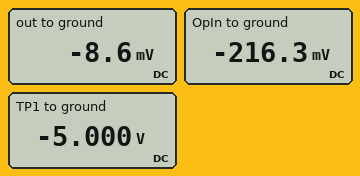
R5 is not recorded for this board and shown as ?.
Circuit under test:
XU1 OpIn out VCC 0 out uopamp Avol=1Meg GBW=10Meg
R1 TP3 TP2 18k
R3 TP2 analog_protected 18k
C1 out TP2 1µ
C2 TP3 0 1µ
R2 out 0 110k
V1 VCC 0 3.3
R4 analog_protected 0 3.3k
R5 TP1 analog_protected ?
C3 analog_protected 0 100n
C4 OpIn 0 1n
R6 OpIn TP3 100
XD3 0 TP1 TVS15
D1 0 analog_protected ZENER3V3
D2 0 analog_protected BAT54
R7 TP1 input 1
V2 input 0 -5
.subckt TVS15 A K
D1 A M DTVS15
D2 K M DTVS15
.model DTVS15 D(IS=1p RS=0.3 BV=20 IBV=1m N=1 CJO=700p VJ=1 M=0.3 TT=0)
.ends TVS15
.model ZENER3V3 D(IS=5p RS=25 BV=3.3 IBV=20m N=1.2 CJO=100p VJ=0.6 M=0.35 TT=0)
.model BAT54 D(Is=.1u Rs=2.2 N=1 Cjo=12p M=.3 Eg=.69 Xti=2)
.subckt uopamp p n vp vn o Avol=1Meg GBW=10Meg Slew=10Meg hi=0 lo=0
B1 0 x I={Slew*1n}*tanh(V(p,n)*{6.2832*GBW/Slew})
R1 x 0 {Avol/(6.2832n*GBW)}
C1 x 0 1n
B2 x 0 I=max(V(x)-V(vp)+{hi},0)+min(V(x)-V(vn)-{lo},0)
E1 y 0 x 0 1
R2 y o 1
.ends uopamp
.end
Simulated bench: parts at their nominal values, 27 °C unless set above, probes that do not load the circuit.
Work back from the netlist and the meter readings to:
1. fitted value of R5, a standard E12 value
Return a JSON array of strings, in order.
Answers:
["10 kΩ"]
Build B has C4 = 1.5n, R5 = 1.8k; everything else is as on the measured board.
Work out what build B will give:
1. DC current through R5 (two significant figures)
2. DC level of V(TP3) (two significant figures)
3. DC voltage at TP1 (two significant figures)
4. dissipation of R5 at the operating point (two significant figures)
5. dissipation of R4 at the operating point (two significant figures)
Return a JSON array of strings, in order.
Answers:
["2.6 mA", "-270 mV", "-5.0 V", "12 mW", "22 µW"]
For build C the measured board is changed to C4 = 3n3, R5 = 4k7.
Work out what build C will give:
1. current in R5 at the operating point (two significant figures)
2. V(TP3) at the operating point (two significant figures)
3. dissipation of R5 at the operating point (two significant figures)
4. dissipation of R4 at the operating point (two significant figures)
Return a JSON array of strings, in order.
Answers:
["1.0 mA", "-240 mV", "4.8 mW", "17 µW"]
